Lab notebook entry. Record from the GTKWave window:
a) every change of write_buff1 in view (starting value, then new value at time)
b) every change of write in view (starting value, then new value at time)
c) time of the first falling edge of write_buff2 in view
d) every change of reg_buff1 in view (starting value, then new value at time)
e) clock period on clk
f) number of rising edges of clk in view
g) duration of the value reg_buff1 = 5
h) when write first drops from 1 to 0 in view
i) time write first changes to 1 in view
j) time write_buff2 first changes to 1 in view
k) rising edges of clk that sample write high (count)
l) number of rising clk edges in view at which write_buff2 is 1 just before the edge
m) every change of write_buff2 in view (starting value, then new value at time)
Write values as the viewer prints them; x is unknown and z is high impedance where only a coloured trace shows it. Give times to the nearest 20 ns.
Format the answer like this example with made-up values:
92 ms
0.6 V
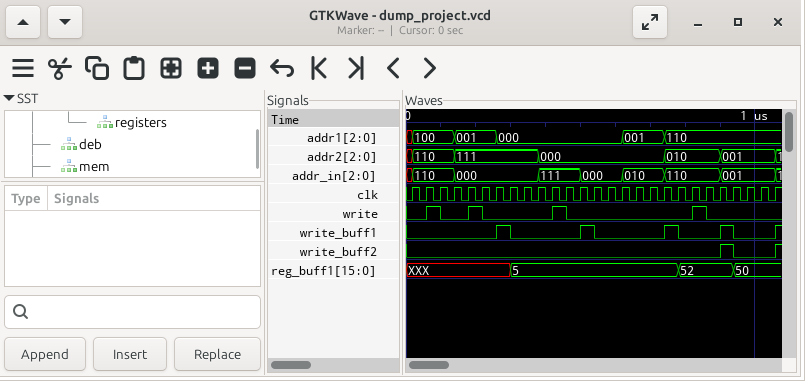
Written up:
0, 1 at 260 ns, 0 at 300 ns, 1 at 500 ns, 0 at 540 ns, 1 at 740 ns, 0 at 780 ns, 1 at 900 ns, 0 at 940 ns, 1 at 1060 ns
0, 1 at 60 ns, 0 at 100 ns, 1 at 180 ns, 0 at 220 ns, 1 at 420 ns, 0 at 460 ns, 1 at 820 ns, 0 at 860 ns
940 ns
XXX, 5 at 300 ns, 52 at 780 ns, 50 at 940 ns
40 ns
27
480 ns
100 ns
60 ns
900 ns
4
1
0, 1 at 900 ns, 0 at 940 ns, 1 at 1060 ns
